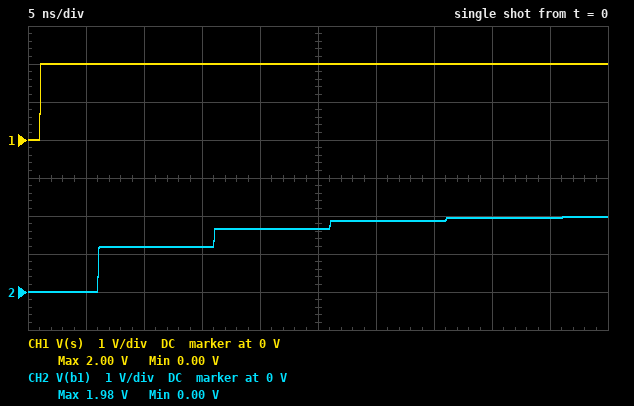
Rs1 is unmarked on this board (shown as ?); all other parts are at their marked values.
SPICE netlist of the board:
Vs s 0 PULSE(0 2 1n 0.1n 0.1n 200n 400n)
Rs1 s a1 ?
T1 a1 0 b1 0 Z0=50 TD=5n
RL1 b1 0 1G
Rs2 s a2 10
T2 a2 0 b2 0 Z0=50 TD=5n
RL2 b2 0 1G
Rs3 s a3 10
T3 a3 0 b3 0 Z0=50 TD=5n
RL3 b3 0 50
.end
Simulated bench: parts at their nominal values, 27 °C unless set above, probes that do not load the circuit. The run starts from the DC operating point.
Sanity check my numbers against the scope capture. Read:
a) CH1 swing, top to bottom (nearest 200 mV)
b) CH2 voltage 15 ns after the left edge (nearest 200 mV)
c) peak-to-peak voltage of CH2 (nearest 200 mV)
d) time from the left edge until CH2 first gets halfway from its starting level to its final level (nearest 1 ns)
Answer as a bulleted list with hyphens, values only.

- 2.0 V
- 1.2 V
- 2.0 V
- 6 ns
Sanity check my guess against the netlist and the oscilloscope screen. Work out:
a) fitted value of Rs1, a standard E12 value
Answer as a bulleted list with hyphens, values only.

- 120 Ω
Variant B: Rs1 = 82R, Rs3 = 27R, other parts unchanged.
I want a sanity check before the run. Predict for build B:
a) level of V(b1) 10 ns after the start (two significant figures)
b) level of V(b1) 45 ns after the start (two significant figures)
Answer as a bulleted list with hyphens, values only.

- 1.5 V
- 2.0 V
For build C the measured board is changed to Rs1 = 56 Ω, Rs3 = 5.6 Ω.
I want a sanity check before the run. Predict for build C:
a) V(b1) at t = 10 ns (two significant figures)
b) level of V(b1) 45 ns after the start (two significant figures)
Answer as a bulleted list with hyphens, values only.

- 1.9 V
- 2.0 V
